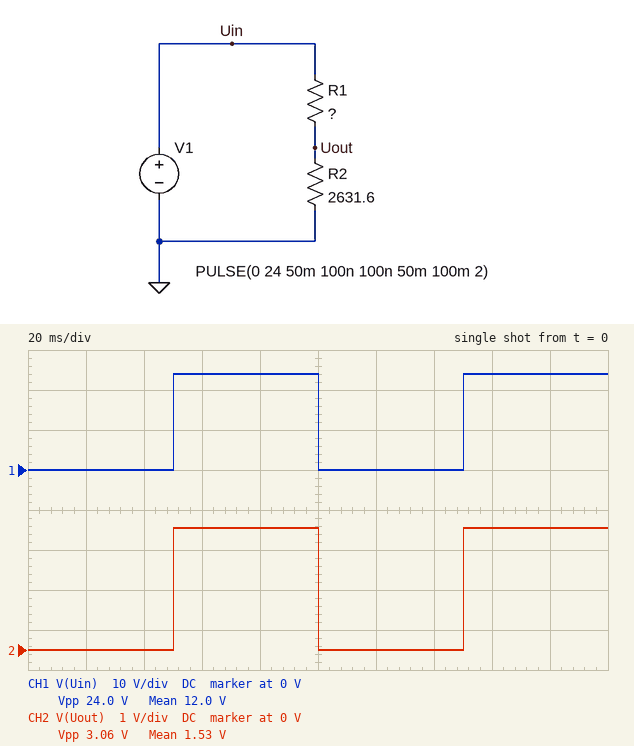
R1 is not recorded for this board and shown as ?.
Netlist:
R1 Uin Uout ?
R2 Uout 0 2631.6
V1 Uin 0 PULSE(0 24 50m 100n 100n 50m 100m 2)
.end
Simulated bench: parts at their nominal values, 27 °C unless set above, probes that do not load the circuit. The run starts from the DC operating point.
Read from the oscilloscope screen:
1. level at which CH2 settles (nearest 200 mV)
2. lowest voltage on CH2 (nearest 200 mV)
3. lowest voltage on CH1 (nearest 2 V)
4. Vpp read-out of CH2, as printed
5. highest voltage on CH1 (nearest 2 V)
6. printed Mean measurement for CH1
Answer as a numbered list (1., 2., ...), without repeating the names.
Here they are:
1. 3.0 V
2. 0 V
3. 0 V
4. 3.06 V
5. 24 V
6. 12.0 V
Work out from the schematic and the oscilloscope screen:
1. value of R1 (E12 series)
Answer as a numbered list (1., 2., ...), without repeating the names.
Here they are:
1. 18 kΩ
